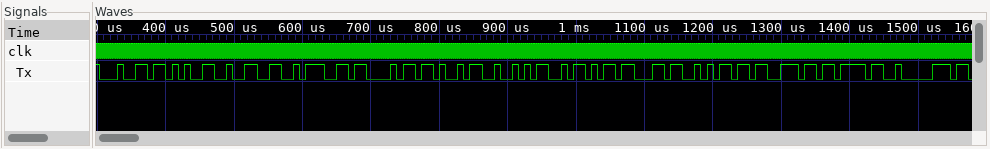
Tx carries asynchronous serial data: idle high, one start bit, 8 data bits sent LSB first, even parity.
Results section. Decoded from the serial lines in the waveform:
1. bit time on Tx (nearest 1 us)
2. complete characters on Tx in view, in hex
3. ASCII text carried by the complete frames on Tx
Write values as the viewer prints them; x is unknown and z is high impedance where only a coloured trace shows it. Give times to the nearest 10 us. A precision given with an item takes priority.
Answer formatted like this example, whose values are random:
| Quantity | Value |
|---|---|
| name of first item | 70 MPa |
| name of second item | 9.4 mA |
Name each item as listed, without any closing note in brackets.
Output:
| Quantity | Value |
|---|---|
| bit time on Tx | 9 us |
| complete characters on Tx in view, in hex | 64, 65, 66, 67, 68, 69, 6A, 6B, 6C, 6D, 6E, 6F, 70 |
| ASCII text carried by the complete frames on Tx | "defghijklmnop" |
